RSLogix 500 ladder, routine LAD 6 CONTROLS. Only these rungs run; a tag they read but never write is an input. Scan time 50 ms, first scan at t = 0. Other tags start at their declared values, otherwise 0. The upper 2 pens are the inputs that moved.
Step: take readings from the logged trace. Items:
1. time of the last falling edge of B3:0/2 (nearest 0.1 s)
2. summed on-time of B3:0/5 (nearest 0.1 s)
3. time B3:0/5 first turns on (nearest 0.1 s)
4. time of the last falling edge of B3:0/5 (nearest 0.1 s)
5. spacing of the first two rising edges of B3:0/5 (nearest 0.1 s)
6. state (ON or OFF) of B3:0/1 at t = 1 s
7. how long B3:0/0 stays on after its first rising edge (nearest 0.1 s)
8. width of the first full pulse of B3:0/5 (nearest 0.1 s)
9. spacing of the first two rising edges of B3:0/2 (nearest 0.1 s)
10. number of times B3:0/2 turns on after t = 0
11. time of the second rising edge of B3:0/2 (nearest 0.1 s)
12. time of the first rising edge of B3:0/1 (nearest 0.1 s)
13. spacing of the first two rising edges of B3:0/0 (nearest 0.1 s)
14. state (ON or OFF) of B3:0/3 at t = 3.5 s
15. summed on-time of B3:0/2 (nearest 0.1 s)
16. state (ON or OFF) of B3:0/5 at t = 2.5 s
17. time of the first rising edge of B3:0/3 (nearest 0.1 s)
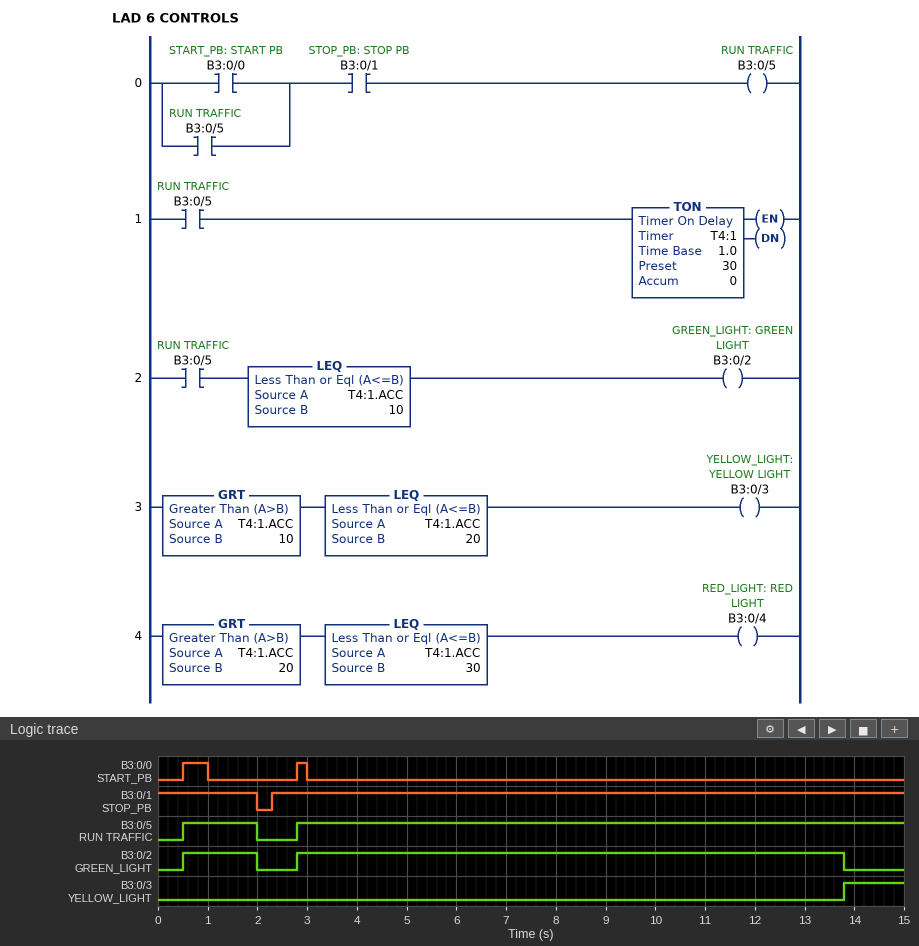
13.8 s
13.7 s
0.5 s
2.0 s
2.3 s
ON
0.5 s
1.5 s
2.3 s
2
2.8 s
2.3 s
2.3 s
OFF
12.5 s
OFF
13.8 s
